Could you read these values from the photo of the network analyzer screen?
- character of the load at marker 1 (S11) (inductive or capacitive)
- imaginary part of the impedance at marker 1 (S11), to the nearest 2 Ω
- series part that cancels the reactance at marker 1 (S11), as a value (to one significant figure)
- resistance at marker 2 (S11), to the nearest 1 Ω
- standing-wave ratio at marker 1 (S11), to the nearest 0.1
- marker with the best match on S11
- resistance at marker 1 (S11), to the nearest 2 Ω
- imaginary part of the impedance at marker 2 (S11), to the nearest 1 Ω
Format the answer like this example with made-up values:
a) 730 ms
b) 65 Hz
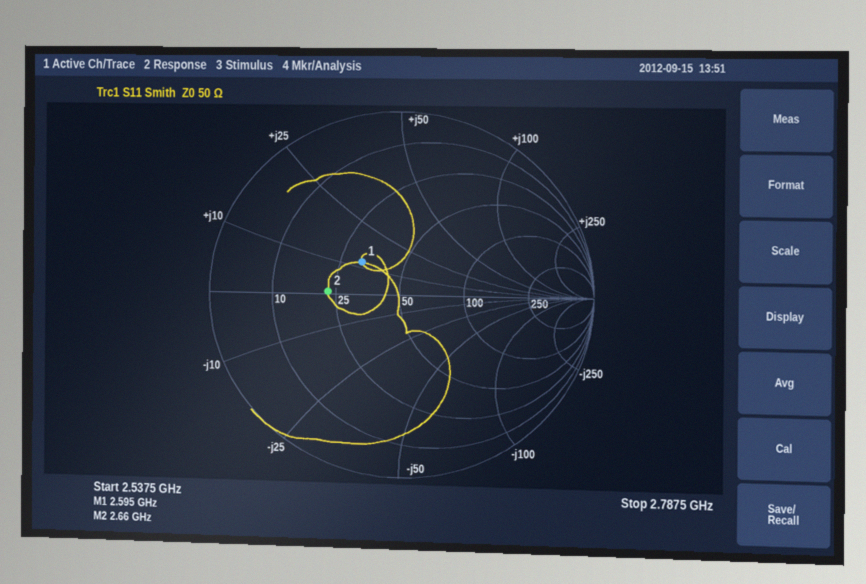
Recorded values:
a) inductive
b) +12 Ω
c) 5 pF
d) 23 Ω
e) 1.7
f) marker 1
g) 32 Ω
h) +1 Ω
